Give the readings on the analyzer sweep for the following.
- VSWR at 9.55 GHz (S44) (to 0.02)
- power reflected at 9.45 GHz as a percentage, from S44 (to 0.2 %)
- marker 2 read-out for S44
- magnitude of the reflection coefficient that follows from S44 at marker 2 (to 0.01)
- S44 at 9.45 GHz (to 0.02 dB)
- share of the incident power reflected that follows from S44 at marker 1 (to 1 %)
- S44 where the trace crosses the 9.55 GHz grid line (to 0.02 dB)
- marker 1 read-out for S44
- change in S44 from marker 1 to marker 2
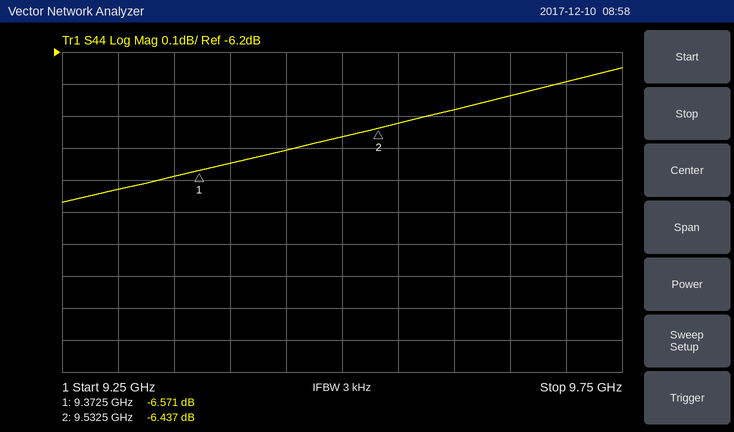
2.82
22.4 %
-6.437 dB
0.48
-6.50 dB
22 %
-6.42 dB
-6.571 dB
0.134 dB
